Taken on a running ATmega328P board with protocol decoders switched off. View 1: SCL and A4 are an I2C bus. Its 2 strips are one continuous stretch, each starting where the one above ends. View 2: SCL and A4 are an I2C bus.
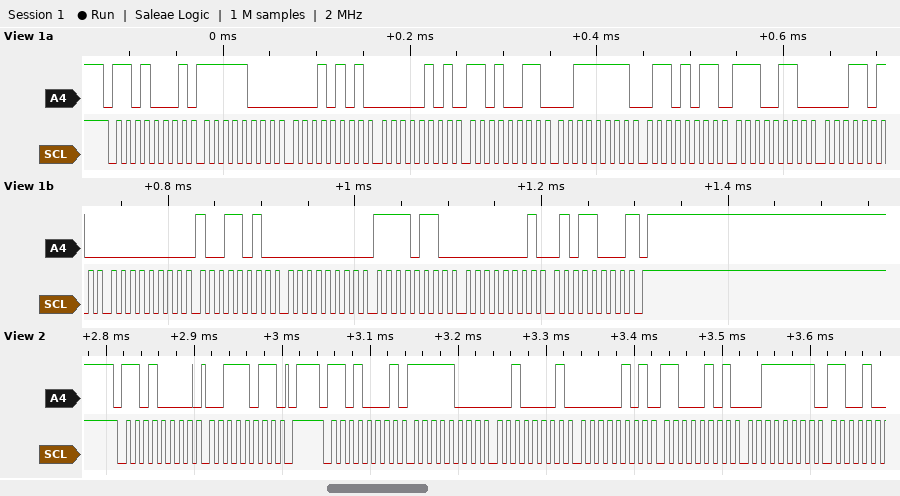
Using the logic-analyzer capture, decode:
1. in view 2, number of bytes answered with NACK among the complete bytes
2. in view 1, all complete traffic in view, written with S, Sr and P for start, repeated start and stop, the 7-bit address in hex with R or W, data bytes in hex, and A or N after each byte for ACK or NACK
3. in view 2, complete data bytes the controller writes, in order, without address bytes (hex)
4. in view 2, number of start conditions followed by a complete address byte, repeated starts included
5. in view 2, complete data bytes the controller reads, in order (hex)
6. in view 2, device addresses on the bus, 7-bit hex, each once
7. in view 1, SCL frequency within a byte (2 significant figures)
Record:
0
S 68R A F8 A 15 A 05 A D3 A 3F A 6B A E6 A 1A A 00 A 9A A 00 A F6 A 01 A 58 N P
3B
2
F8 21 05 C5 3F
0x68
100 kHz
